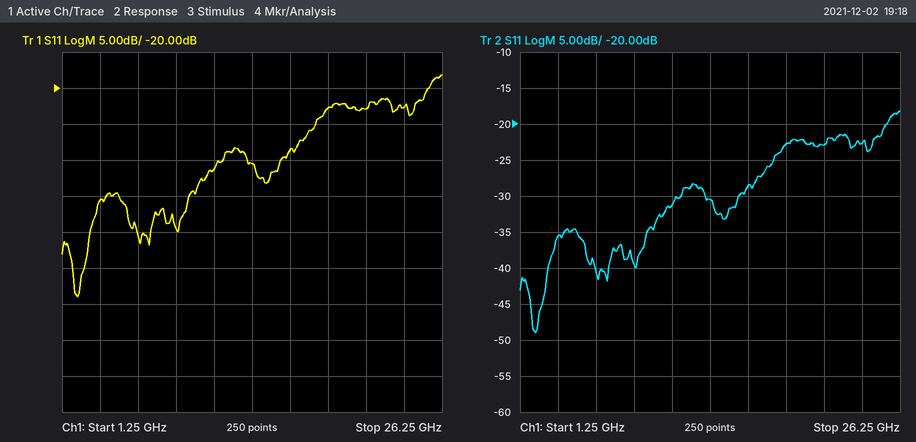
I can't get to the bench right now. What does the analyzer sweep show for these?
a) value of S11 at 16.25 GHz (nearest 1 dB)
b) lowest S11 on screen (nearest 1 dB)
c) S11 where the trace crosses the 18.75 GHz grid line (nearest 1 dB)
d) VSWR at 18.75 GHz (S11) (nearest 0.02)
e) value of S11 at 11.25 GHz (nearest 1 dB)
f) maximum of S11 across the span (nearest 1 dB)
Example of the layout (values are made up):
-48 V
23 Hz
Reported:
-29 dB
-49 dB
-23 dB
1.16
-31 dB
-18 dB
